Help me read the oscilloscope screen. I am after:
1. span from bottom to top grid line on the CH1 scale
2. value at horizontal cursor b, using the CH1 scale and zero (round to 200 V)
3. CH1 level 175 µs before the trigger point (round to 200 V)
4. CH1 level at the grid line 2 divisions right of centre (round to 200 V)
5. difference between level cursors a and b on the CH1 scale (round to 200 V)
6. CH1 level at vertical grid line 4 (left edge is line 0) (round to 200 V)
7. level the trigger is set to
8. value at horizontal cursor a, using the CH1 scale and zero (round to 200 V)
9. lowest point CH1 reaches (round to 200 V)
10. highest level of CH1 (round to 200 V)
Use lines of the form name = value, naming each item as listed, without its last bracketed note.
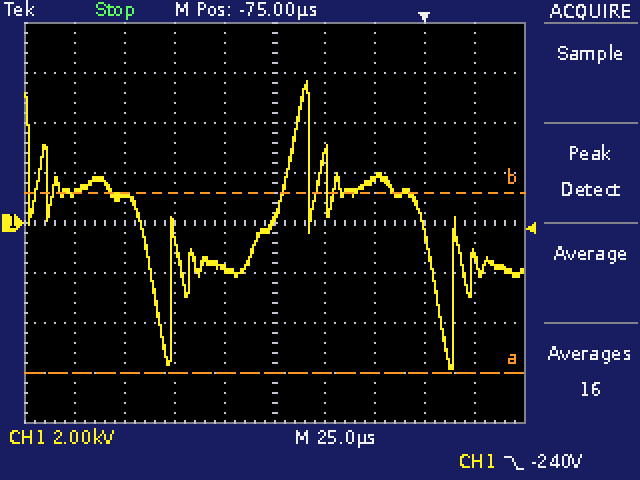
span from bottom to top grid line on the CH1 scale = 16 kV
value at horizontal cursor b, using the CH1 scale and zero = 1.2 kV
CH1 level 175 µs before the trigger point = 1.2 kV
CH1 level at the grid line 2 divisions right of centre = 1.8 kV
difference between level cursors a and b on the CH1 scale = 7.2 kV
CH1 level at vertical grid line 4 (left edge is line 0) = -1.8 kV
level the trigger is set to = -240 V
value at horizontal cursor a, using the CH1 scale and zero = -6.0 kV
lowest point CH1 reaches = -5.8 kV
highest level of CH1 = 5.6 kV
